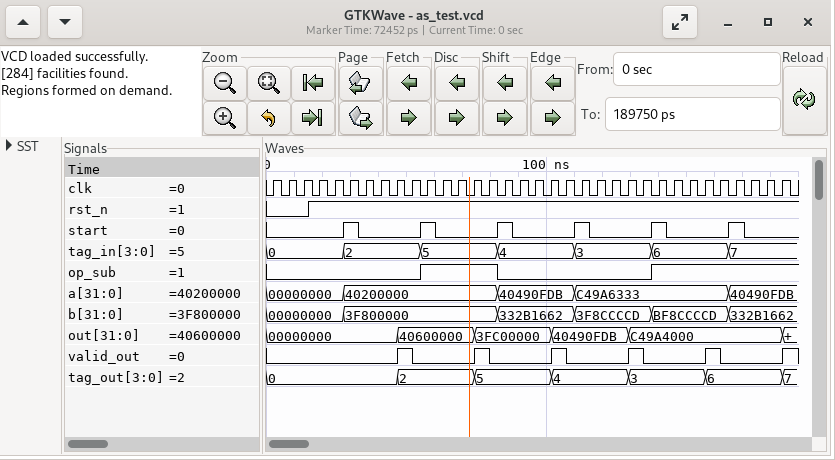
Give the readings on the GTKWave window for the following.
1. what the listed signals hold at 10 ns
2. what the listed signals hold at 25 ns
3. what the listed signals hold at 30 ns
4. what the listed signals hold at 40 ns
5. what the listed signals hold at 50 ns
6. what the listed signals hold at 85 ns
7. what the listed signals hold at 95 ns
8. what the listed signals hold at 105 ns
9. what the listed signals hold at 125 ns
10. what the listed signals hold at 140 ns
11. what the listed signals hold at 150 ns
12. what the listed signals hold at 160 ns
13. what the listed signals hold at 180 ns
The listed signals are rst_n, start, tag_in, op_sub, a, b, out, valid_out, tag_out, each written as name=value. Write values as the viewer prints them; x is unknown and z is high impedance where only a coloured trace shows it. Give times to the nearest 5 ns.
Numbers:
rst_n=0, start=0, tag_in=0, op_sub=0, a=00000000, b=00000000, out=00000000, valid_out=0, tag_out=0
rst_n=1, start=0, tag_in=0, op_sub=0, a=00000000, b=00000000, out=00000000, valid_out=0, tag_out=0
rst_n=1, start=1, tag_in=2, op_sub=0, a=40200000, b=3F800000, out=00000000, valid_out=0, tag_out=0
rst_n=1, start=0, tag_in=2, op_sub=0, a=40200000, b=3F800000, out=00000000, valid_out=0, tag_out=0
rst_n=1, start=0, tag_in=2, op_sub=0, a=40200000, b=3F800000, out=40600000, valid_out=1, tag_out=2
rst_n=1, start=1, tag_in=4, op_sub=0, a=40490FDB, b=332B1662, out=3FC00000, valid_out=0, tag_out=5
rst_n=1, start=0, tag_in=4, op_sub=0, a=40490FDB, b=332B1662, out=3FC00000, valid_out=0, tag_out=5
rst_n=1, start=0, tag_in=4, op_sub=0, a=40490FDB, b=332B1662, out=40490FDB, valid_out=1, tag_out=4
rst_n=1, start=0, tag_in=3, op_sub=0, a=C49A6333, b=3F8CCCCD, out=40490FDB, valid_out=0, tag_out=4
rst_n=1, start=1, tag_in=6, op_sub=1, a=C49A6333, b=BF8CCCCD, out=C49A4000, valid_out=0, tag_out=3
rst_n=1, start=0, tag_in=6, op_sub=1, a=C49A6333, b=BF8CCCCD, out=C49A4000, valid_out=0, tag_out=3
rst_n=1, start=0, tag_in=6, op_sub=1, a=C49A6333, b=BF8CCCCD, out=C49A4000, valid_out=1, tag_out=6
rst_n=1, start=0, tag_in=7, op_sub=1, a=40490FDB, b=332B1662, out=C49A4000, valid_out=0, tag_out=6
